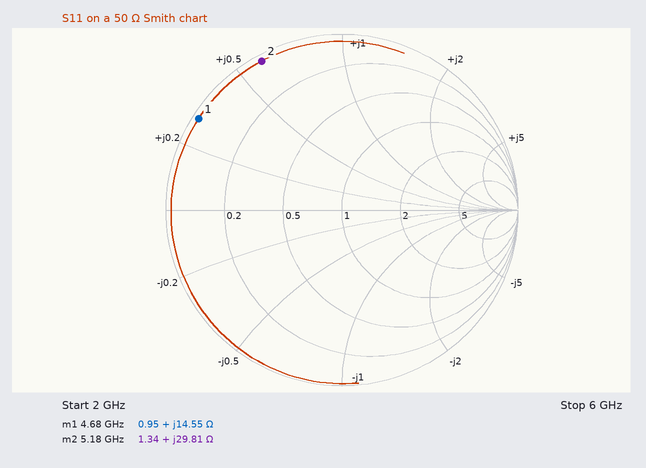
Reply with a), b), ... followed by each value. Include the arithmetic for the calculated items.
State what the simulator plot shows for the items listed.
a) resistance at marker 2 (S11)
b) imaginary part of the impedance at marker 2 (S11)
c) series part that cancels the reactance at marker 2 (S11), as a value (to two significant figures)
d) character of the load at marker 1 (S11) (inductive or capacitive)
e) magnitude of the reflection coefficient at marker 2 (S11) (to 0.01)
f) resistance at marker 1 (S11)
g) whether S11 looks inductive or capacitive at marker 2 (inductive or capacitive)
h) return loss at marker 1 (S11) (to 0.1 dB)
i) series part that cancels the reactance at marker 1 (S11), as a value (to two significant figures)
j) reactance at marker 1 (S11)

a) 1.34 Ω
b) +29.81 Ω
c) C = 1/(2π × 5.18 GHz × 29.81 Ω) ≈ 1.0 pF
d) inductive
e) 0.96
f) 0.95 Ω
g) inductive
h) 0.3 dB
i) C = 1/(2π × 4.68 GHz × 14.55 Ω) ≈ 2.3 pF
j) +14.55 Ω
